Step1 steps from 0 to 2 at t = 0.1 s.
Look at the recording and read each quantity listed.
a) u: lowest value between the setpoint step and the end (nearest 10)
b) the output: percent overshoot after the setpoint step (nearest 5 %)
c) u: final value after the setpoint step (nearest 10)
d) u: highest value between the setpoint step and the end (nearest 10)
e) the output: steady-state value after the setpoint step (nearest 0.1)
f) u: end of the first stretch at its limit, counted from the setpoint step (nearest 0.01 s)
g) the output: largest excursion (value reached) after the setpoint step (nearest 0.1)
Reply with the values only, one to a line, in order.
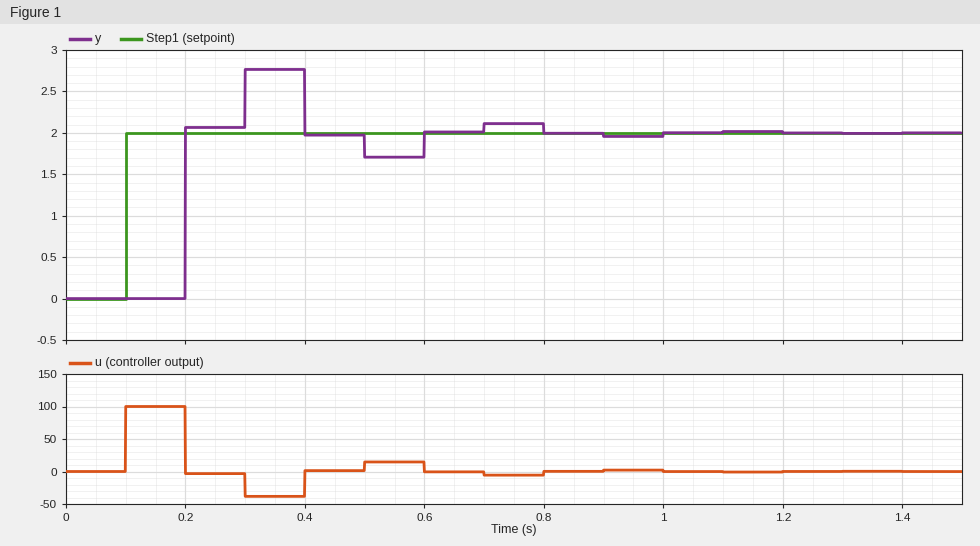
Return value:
-40
40 %
0
100
2.0
0.10 s
2.8
